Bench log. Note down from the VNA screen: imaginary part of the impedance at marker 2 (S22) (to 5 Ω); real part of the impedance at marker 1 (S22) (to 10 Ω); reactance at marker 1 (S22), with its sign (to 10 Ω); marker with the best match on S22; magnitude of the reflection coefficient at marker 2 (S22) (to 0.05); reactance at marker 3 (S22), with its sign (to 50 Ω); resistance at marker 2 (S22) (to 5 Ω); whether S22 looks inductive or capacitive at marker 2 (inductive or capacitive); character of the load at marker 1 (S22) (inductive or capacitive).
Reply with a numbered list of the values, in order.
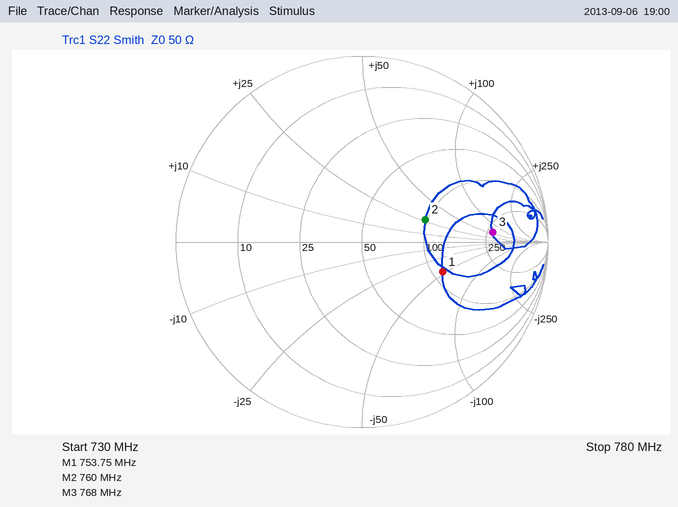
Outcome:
1. +25 Ω
2. 110 Ω
3. -50 Ω
4. marker 2
5. 0.35
6. +50 Ω
7. 95 Ω
8. inductive
9. capacitive
